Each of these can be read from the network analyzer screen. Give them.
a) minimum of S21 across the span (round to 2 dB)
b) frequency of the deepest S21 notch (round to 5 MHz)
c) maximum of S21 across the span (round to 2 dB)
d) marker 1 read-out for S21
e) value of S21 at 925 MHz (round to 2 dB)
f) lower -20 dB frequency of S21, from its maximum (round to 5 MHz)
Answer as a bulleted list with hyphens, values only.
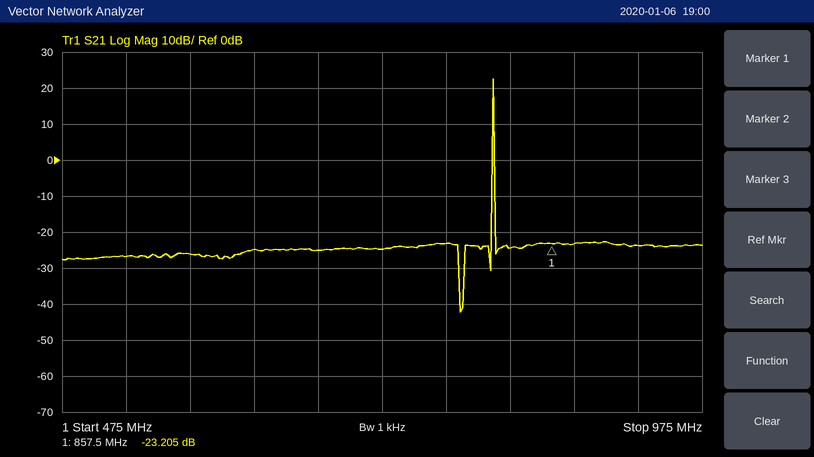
- -42 dB
- 785 MHz
- 22 dB
- -23.205 dB
- -24 dB
- 810 MHz
